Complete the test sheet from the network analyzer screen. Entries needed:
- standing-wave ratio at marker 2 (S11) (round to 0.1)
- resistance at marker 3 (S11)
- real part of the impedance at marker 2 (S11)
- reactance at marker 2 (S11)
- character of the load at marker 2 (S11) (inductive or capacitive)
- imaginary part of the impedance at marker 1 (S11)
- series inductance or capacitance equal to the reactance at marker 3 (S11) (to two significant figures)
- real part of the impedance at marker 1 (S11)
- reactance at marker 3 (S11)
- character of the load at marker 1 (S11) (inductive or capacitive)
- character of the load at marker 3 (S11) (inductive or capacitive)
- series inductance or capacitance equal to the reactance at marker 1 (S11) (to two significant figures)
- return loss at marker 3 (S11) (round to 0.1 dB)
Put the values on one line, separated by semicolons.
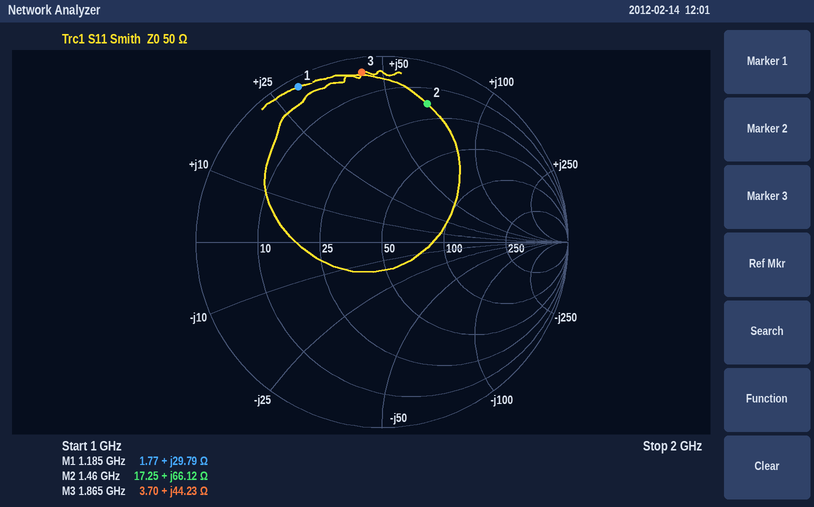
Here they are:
8.2; 3.70 Ω; 17.25 Ω; +66.12 Ω; inductive; +29.79 Ω; 3.8 nH; 1.77 Ω; +44.23 Ω; inductive; inductive; 4.0 nH; 0.7 dB
